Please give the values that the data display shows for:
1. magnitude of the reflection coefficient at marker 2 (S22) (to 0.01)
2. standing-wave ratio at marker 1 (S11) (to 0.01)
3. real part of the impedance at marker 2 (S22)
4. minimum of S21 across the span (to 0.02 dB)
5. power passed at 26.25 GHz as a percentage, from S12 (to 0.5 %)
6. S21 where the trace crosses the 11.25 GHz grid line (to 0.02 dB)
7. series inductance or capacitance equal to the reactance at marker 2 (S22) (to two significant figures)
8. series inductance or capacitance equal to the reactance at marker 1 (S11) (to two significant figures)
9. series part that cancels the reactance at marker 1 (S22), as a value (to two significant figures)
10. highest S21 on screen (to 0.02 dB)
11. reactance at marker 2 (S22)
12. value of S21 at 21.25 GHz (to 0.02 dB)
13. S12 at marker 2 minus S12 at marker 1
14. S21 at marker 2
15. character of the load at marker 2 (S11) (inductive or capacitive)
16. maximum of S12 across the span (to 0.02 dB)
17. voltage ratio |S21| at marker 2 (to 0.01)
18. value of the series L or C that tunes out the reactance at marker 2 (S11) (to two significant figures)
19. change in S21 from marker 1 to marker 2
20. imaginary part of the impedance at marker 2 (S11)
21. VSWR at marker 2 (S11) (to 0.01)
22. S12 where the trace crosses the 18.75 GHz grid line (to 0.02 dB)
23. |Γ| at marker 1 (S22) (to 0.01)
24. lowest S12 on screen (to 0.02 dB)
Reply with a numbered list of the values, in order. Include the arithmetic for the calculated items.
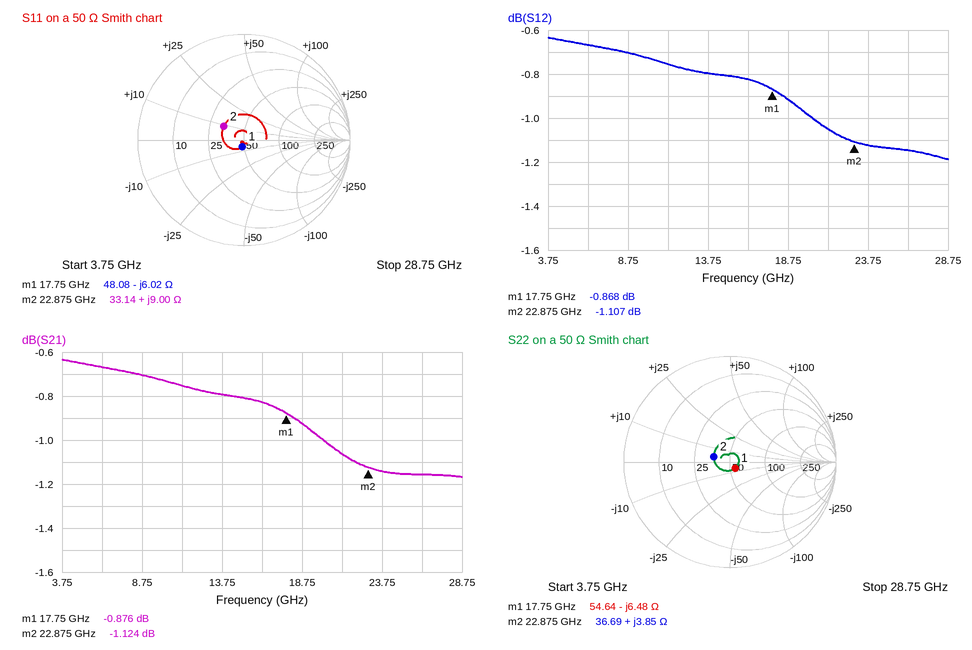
1. 0.16
2. 1.14
3. 36.69 Ω
4. -1.16 dB
5. 10^(-1.14/10) ≈ 76.9 %, so 77.0 % to the nearest 0.5 %
6. -0.76 dB
7. L = 3.85 Ω/(2π × 22.875 GHz) ≈ 27 pH
8. C = 1/(2π × 17.75 GHz × 6.02 Ω) ≈ 1.5 pF
9. L = 6.48 Ω/(2π × 17.75 GHz) ≈ 58 pH
10. -0.64 dB
11. +3.85 Ω
12. -1.06 dB
13. -1.107 − (-0.868) = -0.239 dB
14. -1.124 dB
15. inductive
16. -0.64 dB
17. 10^(-1.124/20) ≈ 0.88
18. C = 1/(2π × 22.875 GHz × 9 Ω) ≈ 773 fF, so 770 fF to two significant figures
19. -1.124 − (-0.876) = -0.248 dB
20. +9.00 Ω
21. 1.59
22. -0.92 dB
23. 0.08
24. -1.18 dB
